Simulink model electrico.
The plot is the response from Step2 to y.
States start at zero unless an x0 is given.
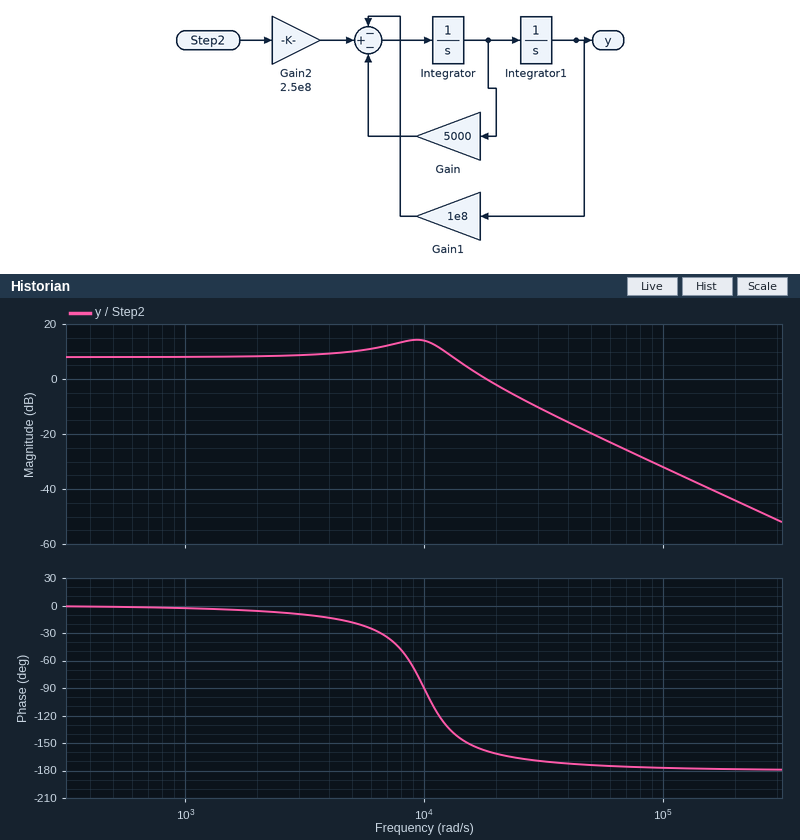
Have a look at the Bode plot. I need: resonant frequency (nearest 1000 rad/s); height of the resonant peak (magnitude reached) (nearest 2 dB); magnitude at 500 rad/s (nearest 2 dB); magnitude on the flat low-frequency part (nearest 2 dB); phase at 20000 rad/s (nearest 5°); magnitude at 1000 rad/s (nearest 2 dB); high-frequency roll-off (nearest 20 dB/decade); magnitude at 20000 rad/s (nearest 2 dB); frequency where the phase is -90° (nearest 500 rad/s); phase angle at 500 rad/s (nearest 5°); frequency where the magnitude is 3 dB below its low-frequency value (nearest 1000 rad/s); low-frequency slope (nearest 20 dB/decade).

9000 rad/s
14 dB
8 dB
8 dB
-160°
8 dB
-40 dB/decade
-2 dB
10000 rad/s
0°
15000 rad/s
0 dB/decade
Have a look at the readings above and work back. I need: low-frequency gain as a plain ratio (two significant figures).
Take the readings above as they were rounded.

2.5
